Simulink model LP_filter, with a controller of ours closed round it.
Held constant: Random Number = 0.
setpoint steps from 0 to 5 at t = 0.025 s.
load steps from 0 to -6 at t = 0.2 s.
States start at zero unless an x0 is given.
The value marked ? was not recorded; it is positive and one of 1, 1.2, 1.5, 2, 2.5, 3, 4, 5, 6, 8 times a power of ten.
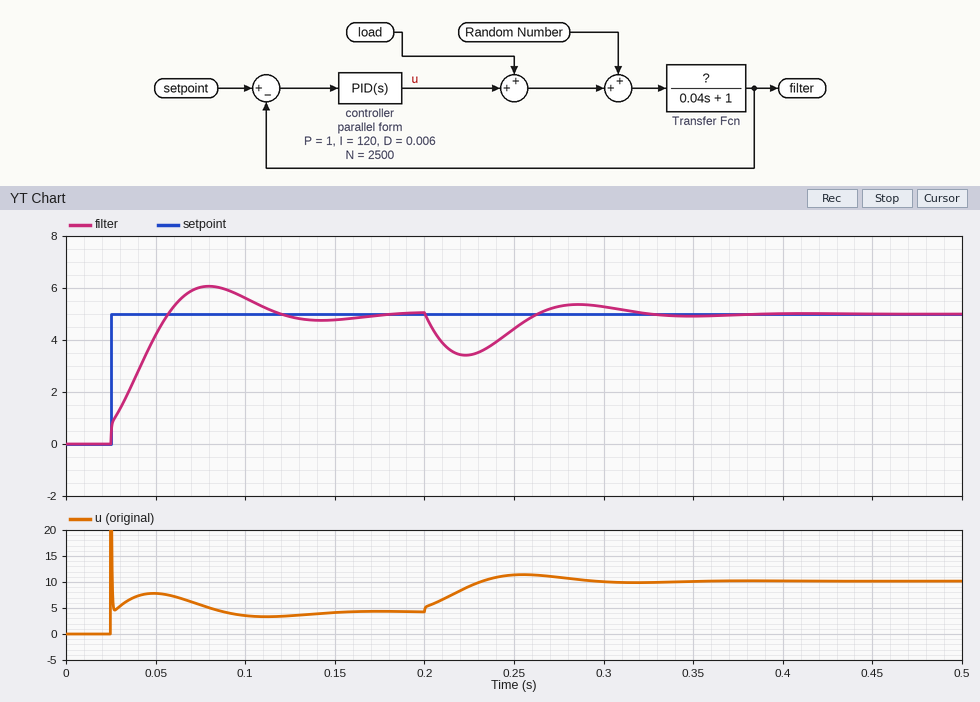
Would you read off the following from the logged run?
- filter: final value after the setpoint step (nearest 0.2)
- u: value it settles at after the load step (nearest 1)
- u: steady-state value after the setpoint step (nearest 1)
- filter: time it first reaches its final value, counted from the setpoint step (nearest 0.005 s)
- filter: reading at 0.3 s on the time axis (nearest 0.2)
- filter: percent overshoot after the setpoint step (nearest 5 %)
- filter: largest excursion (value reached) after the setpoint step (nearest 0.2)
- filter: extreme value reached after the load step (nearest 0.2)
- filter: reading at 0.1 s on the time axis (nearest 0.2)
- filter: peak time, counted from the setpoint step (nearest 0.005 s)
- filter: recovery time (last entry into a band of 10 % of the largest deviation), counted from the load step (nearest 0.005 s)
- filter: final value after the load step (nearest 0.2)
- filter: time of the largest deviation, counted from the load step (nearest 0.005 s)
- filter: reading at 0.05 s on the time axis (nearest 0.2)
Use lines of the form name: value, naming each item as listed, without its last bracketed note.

filter: final value after the setpoint step: 5.0
u: value it settles at after the load step: 10
u: steady-state value after the setpoint step: 4
filter: time it first reaches its final value, counted from the setpoint step: 0.030 s
filter: reading at 0.3 s on the time axis: 5.2
filter: percent overshoot after the setpoint step: 20 %
filter: largest excursion (value reached) after the setpoint step: 6.0
filter: extreme value reached after the load step: 3.4
filter: reading at 0.1 s on the time axis: 5.6
filter: peak time, counted from the setpoint step: 0.055 s
filter: recovery time (last entry into a band of 10 % of the largest deviation), counted from the load step: 0.110 s
filter: final value after the load step: 5.0
filter: time of the largest deviation, counted from the load step: 0.025 s
filter: reading at 0.05 s on the time axis: 4.2
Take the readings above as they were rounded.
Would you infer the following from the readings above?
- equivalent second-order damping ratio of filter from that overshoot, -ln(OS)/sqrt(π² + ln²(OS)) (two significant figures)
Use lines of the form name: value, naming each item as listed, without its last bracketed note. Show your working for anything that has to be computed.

equivalent second-order damping ratio of filter from that overshoot, -ln(OS)/sqrt(π² + ln²(OS)): ln(0.2) = -1.609; 1.609 / sqrt(9.870 + 2.590) = 0.46
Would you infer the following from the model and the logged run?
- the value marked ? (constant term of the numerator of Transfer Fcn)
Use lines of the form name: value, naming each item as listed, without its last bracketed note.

the value marked ?: 1.2
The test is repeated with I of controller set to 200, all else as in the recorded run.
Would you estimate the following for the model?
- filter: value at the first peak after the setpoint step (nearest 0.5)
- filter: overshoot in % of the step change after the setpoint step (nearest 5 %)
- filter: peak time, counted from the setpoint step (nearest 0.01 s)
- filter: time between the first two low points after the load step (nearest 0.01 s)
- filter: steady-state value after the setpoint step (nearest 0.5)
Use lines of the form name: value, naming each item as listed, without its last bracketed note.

filter: value at the first peak after the setpoint step: 6.5
filter: overshoot in % of the step change after the setpoint step: 30 %
filter: peak time, counted from the setpoint step: 0.04 s
filter: time between the first two low points after the load step: 0.09 s
filter: steady-state value after the setpoint step: 5.0
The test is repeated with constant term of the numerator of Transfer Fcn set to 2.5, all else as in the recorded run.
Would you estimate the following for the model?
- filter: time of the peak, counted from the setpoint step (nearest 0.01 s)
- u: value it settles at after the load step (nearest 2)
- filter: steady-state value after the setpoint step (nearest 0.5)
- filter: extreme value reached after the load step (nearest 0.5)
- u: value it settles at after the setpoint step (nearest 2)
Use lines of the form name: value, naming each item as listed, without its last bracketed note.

filter: time of the peak, counted from the setpoint step: 0.04 s
u: value it settles at after the load step: 8
filter: steady-state value after the setpoint step: 5.0
filter: extreme value reached after the load step: 3.0
u: value it settles at after the setpoint step: 2
